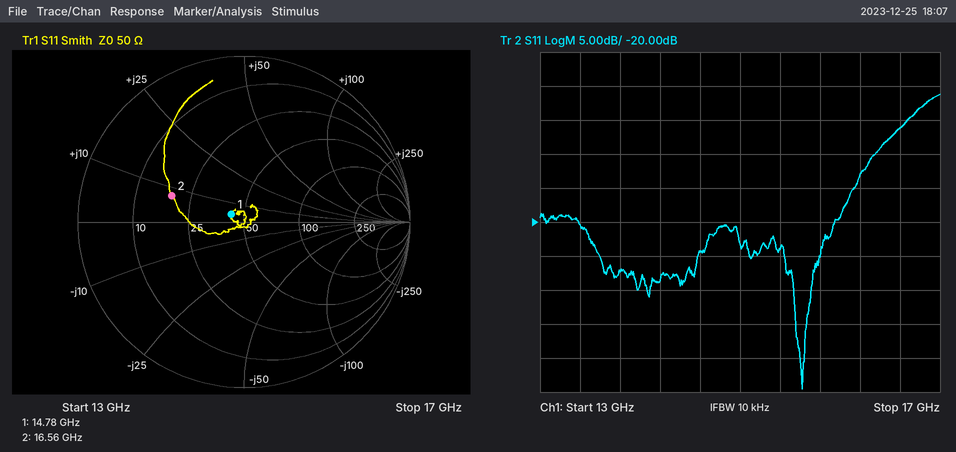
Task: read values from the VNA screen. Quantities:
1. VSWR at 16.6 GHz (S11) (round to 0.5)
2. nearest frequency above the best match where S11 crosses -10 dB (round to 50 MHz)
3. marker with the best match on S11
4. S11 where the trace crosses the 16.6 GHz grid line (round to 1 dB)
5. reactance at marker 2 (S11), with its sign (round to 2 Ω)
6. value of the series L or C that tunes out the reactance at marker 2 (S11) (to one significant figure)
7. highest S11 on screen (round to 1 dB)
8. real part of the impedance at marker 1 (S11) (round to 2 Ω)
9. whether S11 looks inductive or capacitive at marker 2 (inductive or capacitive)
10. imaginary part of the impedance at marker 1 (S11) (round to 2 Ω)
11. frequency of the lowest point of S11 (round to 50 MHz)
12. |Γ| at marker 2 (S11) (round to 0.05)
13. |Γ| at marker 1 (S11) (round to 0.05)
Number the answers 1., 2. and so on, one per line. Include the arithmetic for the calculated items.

1. |Γ| = 10^(-6/20) = 0.5012; VSWR = (1 + 0.5012)/(1 − 0.5012) ≈ 3.0
2. 16.35 GHz
3. marker 1
4. -6 dB
5. +8 Ω
6. C = 1/(2π × 16.56 GHz × 8 Ω) ≈ 1 pF
7. -1 dB
8. 42 Ω
9. inductive
10. +4 Ω
11. 15.60 GHz
12. 0.45
13. 0.10
